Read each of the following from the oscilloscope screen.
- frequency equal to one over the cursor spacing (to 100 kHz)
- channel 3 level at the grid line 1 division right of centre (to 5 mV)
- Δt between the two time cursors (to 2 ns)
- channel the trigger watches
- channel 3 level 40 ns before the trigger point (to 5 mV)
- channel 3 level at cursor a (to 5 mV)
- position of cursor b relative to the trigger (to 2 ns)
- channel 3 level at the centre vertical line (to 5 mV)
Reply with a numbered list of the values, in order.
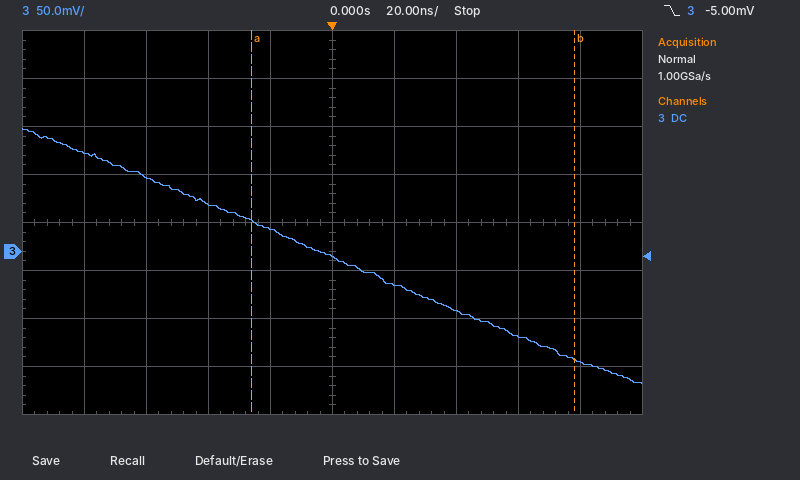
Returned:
1. 9.6 MHz
2. -35 mV
3. 104 ns
4. channel 3
5. 50 mV
6. 30 mV
7. +78 ns
8. -5 mV
